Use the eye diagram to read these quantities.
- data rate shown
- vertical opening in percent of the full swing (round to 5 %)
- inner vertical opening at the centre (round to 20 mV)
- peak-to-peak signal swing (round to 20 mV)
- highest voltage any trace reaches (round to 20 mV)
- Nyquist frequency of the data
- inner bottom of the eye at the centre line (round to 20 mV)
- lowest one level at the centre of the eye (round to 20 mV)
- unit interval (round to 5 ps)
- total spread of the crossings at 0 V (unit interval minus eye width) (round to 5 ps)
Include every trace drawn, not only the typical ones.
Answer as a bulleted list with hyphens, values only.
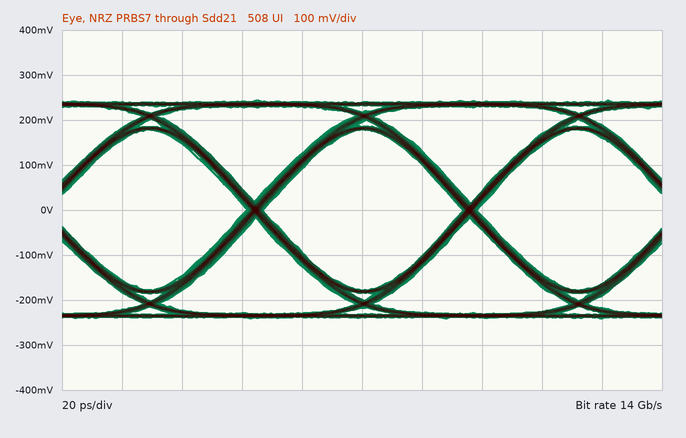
- 14 Gb/s
- 75 %
- 360 mV
- 480 mV
- 240 mV
- 7 GHz
- -180 mV
- 180 mV
- 70 ps
- 5 ps
